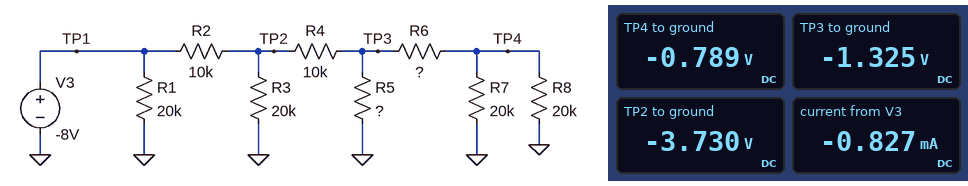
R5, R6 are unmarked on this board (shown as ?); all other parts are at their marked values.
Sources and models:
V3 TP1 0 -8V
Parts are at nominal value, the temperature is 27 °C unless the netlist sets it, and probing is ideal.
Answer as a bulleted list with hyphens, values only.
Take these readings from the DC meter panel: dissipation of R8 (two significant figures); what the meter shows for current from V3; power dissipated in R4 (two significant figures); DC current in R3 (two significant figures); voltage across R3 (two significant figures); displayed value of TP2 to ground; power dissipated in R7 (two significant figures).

- 31 µW
- -0.827 mA
- 580 µW
- 190 µA
- 3.7 V
- -3.730 V
- 31 µW
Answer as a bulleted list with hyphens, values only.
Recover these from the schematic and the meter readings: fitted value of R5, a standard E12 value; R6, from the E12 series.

- 8.2 kΩ
- 6.8 kΩ
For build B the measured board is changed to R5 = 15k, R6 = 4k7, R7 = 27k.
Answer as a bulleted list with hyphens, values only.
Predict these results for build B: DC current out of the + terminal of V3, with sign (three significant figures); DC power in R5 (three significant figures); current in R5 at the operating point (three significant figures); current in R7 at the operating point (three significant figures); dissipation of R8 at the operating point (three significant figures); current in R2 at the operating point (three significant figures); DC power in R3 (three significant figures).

- -812 µA
- 192 µW
- 113 µA
- 44.6 µA
- 72.6 µW
- 412 µA
- 752 µW
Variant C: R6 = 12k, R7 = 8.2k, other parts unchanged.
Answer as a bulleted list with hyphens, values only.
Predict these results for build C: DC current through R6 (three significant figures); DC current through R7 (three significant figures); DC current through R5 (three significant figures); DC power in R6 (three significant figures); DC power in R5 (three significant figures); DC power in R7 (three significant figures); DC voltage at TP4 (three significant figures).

- 75.4 µA
- 53.5 µA
- 164 µA
- 68.3 µW
- 220 µW
- 23.5 µW
- -439 mV
